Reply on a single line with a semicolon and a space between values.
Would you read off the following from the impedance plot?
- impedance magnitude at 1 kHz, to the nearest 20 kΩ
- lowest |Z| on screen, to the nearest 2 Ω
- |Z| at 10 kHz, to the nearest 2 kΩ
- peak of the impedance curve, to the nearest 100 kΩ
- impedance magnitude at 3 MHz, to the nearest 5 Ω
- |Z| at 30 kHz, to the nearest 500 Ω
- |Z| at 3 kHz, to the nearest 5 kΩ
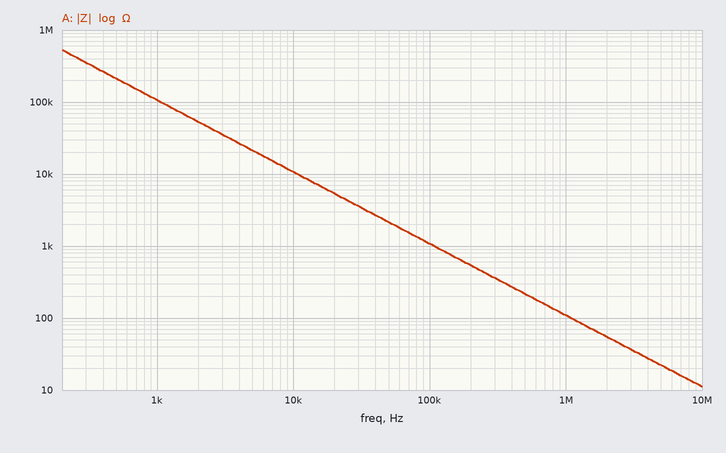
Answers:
100 kΩ; 12 Ω; 10 kΩ; 500 kΩ; 35 Ω; 3.5 kΩ; 35 kΩ
